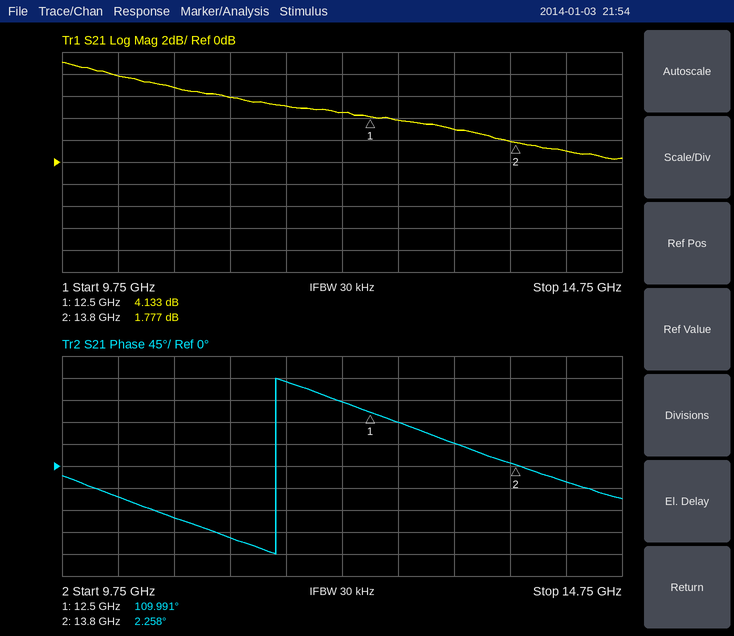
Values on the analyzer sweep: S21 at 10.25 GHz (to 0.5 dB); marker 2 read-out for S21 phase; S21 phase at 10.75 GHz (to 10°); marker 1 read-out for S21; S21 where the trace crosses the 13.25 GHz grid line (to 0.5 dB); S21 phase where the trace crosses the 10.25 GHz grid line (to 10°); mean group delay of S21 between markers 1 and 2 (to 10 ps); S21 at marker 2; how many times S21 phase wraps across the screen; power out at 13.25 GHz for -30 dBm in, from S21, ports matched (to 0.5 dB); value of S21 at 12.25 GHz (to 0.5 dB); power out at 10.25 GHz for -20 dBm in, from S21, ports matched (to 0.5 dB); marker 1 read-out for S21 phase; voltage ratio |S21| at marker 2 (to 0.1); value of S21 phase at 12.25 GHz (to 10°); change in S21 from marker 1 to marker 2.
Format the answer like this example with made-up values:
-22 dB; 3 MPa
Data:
8.0 dB; 2.258°; -110°; 4.133 dB; 3.0 dB; -60°; 230 ps; 1.777 dB; 1; -27.0 dBm; 4.5 dB; -12.0 dBm; 109.991°; 1.2; 130°; -2.356 dB
